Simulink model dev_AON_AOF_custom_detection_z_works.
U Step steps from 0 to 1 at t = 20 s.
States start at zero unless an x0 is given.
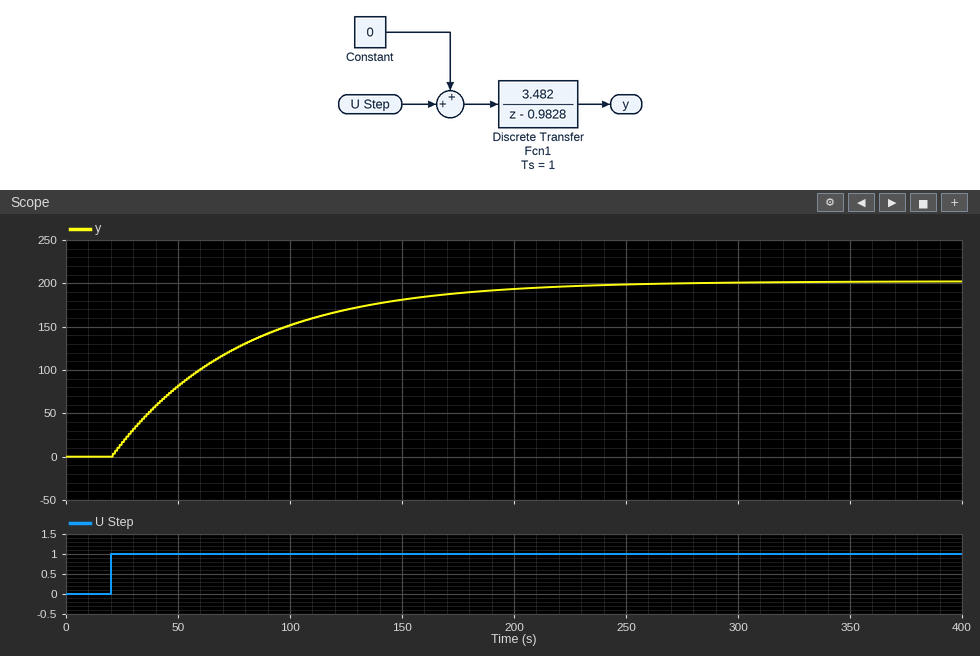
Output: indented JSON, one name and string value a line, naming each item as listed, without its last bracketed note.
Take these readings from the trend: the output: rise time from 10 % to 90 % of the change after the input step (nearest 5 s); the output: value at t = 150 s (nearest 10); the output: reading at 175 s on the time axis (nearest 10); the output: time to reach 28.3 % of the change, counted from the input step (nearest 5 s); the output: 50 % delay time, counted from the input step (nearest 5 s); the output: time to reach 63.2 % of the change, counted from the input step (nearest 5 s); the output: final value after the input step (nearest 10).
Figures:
{
  "the output: rise time from 10 % to 90 % of the change after the input step": "125 s",
  "the output: value at t = 150 s": "180",
  "the output: reading at 175 s on the time axis": "190",
  "the output: time to reach 28.3 % of the change, counted from the input step": "20 s",
  "the output: 50 % delay time, counted from the input step": "40 s",
  "the output: time to reach 63.2 % of the change, counted from the input step": "60 s",
  "the output: final value after the input step": "200"
}
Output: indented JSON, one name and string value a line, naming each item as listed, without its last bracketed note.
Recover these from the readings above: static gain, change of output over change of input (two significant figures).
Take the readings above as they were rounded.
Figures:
{
  "static gain, change of output over change of input": "200"
}
